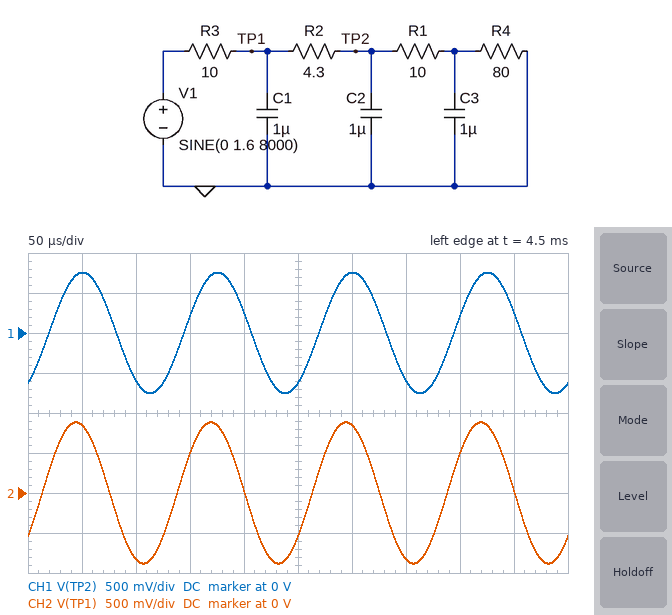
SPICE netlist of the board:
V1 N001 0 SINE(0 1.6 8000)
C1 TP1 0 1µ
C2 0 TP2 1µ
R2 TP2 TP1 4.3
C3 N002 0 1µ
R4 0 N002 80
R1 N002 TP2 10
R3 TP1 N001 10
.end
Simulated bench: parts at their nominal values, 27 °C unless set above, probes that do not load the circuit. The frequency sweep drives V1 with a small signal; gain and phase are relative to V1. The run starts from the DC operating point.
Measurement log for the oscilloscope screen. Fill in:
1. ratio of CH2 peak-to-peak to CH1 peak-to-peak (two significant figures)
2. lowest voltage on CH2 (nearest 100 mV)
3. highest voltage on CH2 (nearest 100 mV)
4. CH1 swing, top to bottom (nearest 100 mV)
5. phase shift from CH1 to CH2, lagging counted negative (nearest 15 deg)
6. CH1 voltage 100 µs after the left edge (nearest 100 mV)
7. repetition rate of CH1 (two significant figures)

1.2
-900 mV
900 mV
1.5 V
15 deg
-600 mV
8.0 kHz
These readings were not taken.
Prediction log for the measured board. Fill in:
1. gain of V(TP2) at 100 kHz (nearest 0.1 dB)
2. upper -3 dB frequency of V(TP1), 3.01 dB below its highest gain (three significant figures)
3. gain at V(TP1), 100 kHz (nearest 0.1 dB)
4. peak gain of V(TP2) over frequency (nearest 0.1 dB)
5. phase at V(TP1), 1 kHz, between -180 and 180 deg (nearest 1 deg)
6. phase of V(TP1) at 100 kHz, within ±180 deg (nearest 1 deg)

-27.4 dB
5.79 kHz
-17.6 dB
-1.3 dB
-8 deg
-67 deg
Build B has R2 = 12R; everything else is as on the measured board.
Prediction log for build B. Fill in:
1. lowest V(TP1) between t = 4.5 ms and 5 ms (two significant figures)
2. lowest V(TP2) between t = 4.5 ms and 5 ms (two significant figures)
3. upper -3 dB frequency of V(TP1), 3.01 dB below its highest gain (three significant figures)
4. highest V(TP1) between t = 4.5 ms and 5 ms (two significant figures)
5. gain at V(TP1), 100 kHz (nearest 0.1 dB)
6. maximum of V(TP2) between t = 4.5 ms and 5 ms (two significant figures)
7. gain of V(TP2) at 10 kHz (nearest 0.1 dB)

-970 mV
-590 mV
6.59 kHz
970 mV
-16.4 dB
590 mV
-10.2 dB
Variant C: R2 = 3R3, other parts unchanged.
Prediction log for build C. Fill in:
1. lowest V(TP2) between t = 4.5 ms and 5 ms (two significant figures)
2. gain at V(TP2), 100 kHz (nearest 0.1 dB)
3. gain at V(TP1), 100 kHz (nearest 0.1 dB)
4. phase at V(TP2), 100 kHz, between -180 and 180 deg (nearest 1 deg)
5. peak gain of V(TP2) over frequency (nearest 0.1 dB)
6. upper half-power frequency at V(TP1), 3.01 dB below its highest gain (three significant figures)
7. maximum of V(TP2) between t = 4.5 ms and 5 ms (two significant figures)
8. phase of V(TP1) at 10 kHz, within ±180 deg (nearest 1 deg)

-780 mV
-26.1 dB
-18.1 dB
-123 deg
-1.2 dB
5.78 kHz
780 mV
-42 deg
